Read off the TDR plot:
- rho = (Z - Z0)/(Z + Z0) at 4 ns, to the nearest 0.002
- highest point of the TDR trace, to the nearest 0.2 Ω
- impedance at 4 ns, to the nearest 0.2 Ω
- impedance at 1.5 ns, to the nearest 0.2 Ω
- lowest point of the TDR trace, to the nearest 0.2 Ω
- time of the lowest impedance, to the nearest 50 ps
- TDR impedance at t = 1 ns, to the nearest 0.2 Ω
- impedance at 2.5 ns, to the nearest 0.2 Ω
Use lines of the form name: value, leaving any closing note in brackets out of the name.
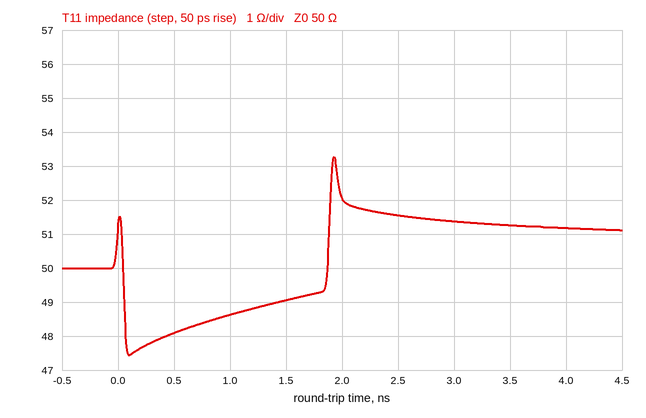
rho = (Z - Z0)/(Z + Z0) at 4 ns, to the nearest 0.002: +0.012
highest point of the TDR trace, to the nearest 0.2 Ω: 53.2 Ω
impedance at 4 ns, to the nearest 0.2 Ω: 51.2 Ω
impedance at 1.5 ns, to the nearest 0.2 Ω: 49.0 Ω
lowest point of the TDR trace, to the nearest 0.2 Ω: 47.4 Ω
time of the lowest impedance, to the nearest 50 ps: 100 ps
TDR impedance at t = 1 ns, to the nearest 0.2 Ω: 48.6 Ω
impedance at 2.5 ns, to the nearest 0.2 Ω: 51.6 Ω
